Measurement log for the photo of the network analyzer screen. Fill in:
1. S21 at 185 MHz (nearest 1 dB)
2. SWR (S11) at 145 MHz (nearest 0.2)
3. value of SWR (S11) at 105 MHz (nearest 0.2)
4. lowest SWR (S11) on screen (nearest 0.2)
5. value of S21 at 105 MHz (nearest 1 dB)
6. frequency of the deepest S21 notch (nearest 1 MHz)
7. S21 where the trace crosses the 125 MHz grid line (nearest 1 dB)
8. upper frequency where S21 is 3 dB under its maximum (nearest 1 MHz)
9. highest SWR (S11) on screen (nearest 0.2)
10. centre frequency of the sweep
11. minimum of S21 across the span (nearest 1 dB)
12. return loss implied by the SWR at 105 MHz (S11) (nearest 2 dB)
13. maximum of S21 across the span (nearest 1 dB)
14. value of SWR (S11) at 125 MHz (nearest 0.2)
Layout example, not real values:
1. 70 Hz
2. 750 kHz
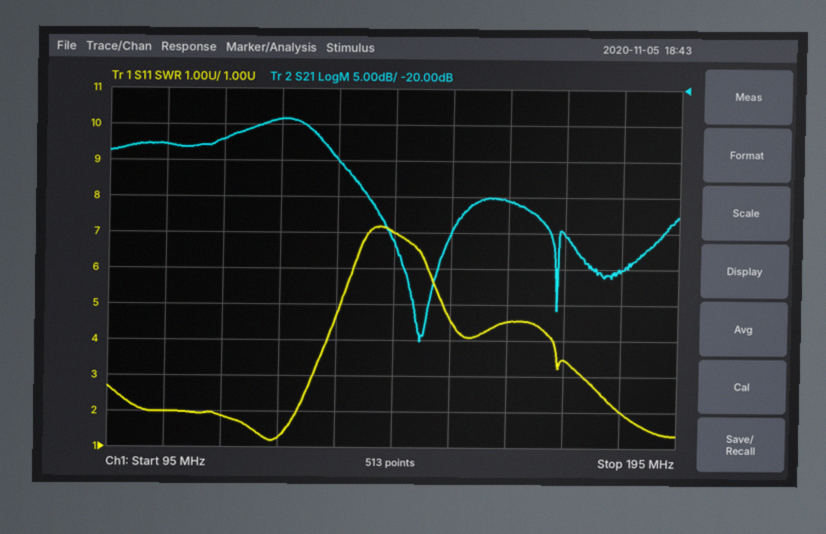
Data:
1. -45 dB
2. 7.0
3. 2.0
4. 1.2
5. -28 dB
6. 150 MHz
7. -24 dB
8. 132 MHz
9. 7.2
10. 145 MHz
11. -55 dB
12. 10 dB
13. -24 dB
14. 1.2
